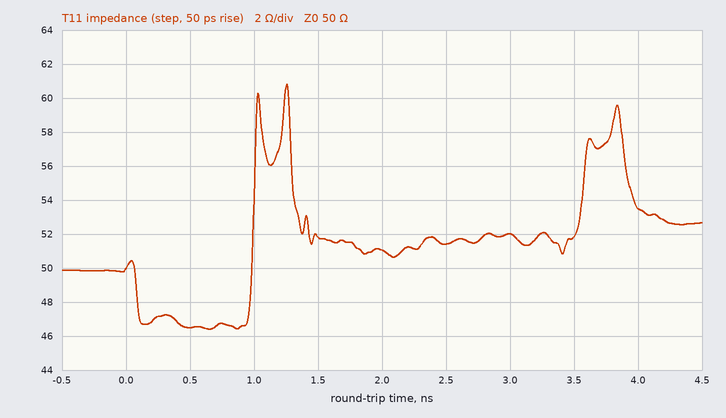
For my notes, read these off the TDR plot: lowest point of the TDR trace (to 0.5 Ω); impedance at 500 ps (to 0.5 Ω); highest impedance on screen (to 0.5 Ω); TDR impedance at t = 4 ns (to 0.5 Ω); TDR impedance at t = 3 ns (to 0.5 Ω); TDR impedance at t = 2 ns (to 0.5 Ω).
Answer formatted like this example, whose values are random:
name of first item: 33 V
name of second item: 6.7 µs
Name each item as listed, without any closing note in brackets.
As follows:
lowest point of the TDR trace: 46.5 Ω
impedance at 500 ps: 46.5 Ω
highest impedance on screen: 61.0 Ω
TDR impedance at t = 4 ns: 53.5 Ω
TDR impedance at t = 3 ns: 52.0 Ω
TDR impedance at t = 2 ns: 51.0 Ω
